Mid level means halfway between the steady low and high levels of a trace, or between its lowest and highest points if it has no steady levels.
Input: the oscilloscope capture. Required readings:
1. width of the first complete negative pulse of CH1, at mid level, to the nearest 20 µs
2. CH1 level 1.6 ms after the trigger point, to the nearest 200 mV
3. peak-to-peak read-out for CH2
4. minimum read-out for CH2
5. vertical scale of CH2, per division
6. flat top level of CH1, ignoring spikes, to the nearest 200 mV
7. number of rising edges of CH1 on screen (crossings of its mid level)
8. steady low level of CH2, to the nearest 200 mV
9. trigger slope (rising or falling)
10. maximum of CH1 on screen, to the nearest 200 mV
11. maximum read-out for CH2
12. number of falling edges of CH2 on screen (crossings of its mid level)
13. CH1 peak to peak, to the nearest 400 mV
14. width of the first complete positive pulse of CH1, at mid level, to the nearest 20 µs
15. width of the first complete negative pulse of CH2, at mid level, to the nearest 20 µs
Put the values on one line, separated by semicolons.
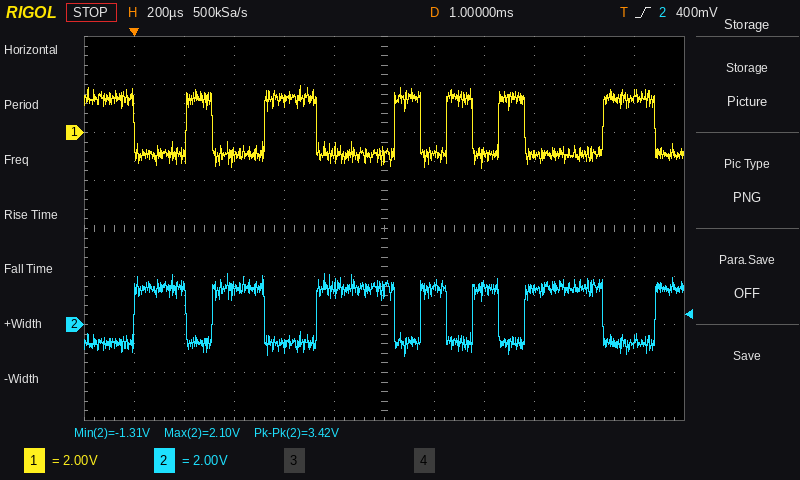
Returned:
200 µs; -1.0 V; 3.42 V; -1.31 V; 2 V; 1.4 V; 6; -800 mV; rising; 2.0 V; 2.10 V; 6; 3.6 V; 100 µs; 100 µs
